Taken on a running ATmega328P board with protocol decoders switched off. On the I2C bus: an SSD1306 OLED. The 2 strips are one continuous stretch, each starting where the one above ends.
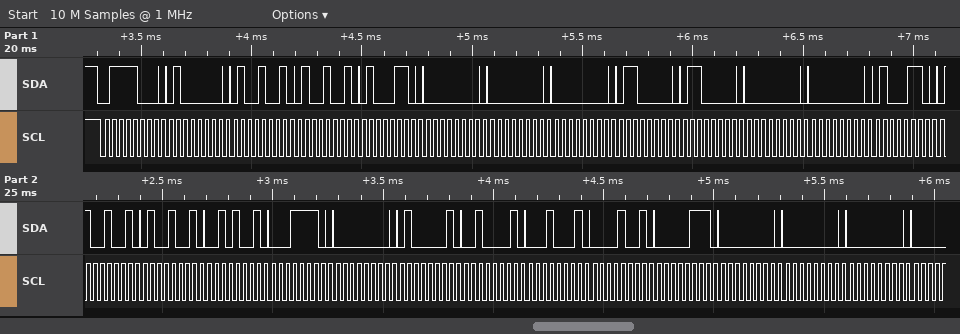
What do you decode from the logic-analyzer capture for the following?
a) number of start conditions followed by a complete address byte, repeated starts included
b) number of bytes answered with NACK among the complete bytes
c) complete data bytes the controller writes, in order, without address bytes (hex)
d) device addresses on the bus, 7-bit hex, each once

1
0
40 49 49 46 00 00 00 60 60 00 00 46 49 49 29 1E 00 41 21 11 09 07 00 00 00
0x3C
